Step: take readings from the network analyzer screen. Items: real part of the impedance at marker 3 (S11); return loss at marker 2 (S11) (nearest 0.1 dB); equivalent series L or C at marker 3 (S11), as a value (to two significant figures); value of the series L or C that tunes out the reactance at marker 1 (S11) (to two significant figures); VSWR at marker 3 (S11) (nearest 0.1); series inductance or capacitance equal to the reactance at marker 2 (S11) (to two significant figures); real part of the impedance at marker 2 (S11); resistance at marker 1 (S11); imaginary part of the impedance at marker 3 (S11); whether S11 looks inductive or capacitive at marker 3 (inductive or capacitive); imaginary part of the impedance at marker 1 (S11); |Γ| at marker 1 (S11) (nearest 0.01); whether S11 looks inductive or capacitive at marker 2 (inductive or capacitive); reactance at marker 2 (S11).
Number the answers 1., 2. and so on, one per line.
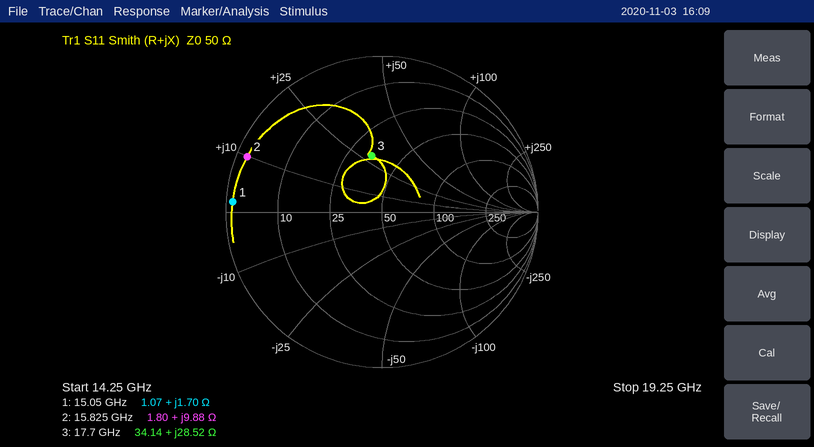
1. 34.14 Ω
2. 0.6 dB
3. 260 pH
4. 6.2 pF
5. 2.2
6. 99 pH
7. 1.80 Ω
8. 1.07 Ω
9. +28.52 Ω
10. inductive
11. +1.70 Ω
12. 0.96
13. inductive
14. +9.88 Ω
